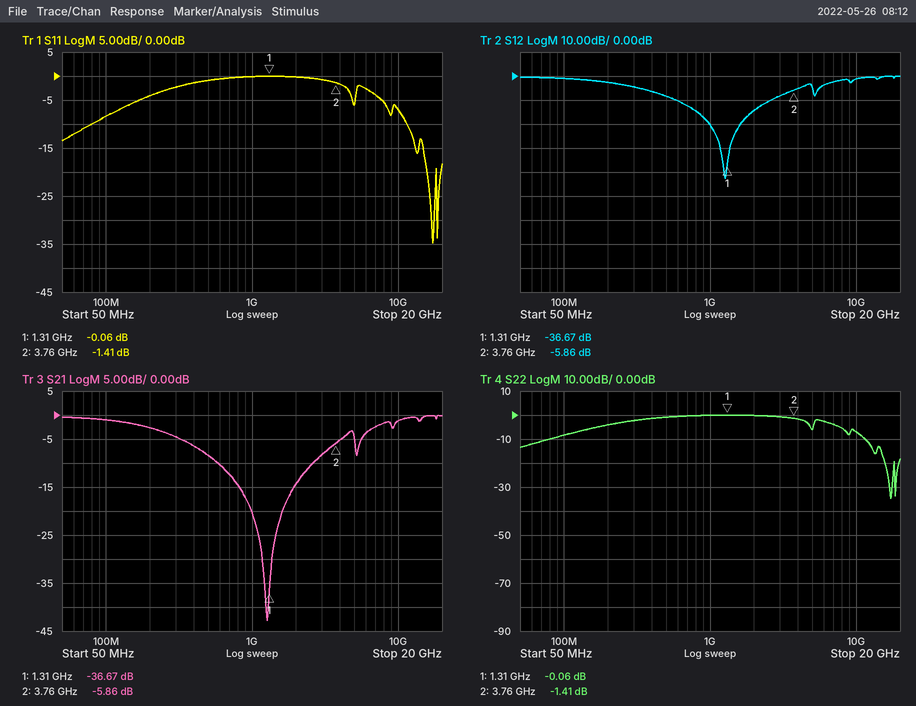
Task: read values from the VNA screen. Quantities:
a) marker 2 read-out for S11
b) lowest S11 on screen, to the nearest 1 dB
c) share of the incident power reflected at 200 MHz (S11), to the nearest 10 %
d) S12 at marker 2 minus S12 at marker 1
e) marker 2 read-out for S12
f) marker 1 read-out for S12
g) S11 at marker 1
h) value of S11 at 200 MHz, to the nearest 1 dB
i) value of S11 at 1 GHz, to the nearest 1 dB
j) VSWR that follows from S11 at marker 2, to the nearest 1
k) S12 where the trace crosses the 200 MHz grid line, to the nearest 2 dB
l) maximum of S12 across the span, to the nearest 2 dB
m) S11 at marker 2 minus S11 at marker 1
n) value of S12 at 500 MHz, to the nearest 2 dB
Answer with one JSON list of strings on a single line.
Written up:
["-1.41 dB", "-35 dB", "40 %", "30.81 dB", "-5.86 dB", "-36.67 dB", "-0.06 dB", "-4 dB", "0 dB", "12", "-2 dB", "0 dB", "-1.35 dB", "-8 dB"]
